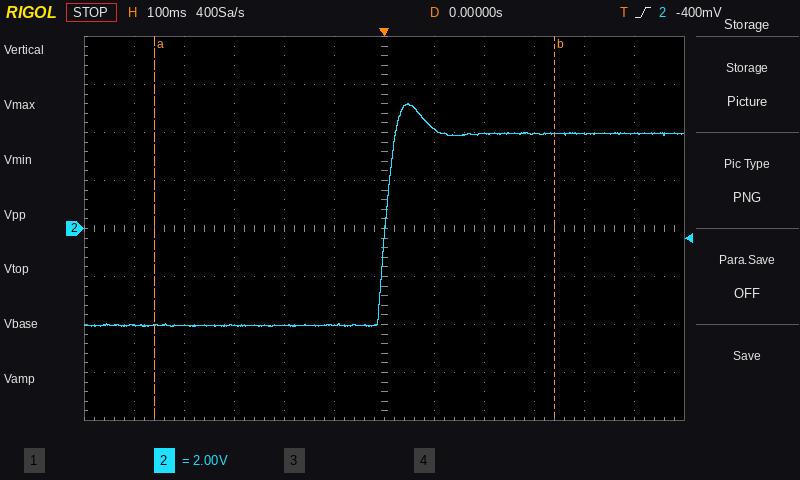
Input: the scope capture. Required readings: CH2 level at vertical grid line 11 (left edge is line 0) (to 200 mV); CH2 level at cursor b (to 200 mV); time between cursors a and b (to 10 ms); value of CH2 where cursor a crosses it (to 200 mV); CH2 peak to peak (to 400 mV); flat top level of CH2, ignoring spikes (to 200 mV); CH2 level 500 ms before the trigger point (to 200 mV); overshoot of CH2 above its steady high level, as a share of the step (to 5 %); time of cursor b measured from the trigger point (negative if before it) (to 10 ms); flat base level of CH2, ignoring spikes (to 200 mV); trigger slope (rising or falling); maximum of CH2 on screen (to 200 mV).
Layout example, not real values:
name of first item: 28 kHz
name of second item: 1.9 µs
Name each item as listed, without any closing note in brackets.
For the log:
CH2 level at vertical grid line 11 (left edge is line 0): 4.0 V
CH2 level at cursor b: 4.0 V
time between cursors a and b: 800 ms
value of CH2 where cursor a crosses it: -4.0 V
CH2 peak to peak: 9.2 V
flat top level of CH2, ignoring spikes: 4.0 V
CH2 level 500 ms before the trigger point: -4.0 V
overshoot of CH2 above its steady high level, as a share of the step: 15 %
time of cursor b measured from the trigger point (negative if before it): +340 ms
flat base level of CH2, ignoring spikes: -4.0 V
trigger slope: rising
maximum of CH2 on screen: 5.2 V
